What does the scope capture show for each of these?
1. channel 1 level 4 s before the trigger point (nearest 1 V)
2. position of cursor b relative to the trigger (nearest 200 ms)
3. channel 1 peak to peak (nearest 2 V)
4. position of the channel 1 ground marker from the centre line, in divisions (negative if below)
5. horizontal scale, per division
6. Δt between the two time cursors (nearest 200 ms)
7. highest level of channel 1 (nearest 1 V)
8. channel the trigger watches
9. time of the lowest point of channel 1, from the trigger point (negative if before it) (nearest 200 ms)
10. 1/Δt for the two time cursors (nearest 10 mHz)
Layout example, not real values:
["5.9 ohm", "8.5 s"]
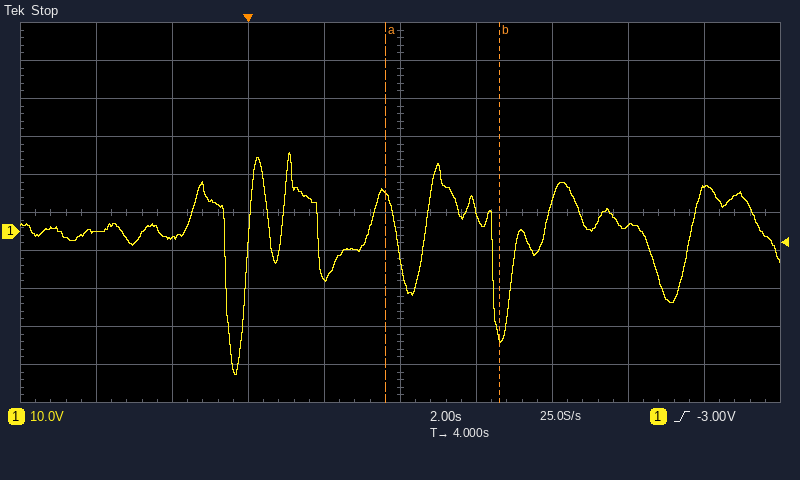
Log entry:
["0 V", "+6.6 s", "58 V", "-0.5 div", "2 s", "3.0 s", "21 V", "channel 1", "-400 ms", "330 mHz"]
